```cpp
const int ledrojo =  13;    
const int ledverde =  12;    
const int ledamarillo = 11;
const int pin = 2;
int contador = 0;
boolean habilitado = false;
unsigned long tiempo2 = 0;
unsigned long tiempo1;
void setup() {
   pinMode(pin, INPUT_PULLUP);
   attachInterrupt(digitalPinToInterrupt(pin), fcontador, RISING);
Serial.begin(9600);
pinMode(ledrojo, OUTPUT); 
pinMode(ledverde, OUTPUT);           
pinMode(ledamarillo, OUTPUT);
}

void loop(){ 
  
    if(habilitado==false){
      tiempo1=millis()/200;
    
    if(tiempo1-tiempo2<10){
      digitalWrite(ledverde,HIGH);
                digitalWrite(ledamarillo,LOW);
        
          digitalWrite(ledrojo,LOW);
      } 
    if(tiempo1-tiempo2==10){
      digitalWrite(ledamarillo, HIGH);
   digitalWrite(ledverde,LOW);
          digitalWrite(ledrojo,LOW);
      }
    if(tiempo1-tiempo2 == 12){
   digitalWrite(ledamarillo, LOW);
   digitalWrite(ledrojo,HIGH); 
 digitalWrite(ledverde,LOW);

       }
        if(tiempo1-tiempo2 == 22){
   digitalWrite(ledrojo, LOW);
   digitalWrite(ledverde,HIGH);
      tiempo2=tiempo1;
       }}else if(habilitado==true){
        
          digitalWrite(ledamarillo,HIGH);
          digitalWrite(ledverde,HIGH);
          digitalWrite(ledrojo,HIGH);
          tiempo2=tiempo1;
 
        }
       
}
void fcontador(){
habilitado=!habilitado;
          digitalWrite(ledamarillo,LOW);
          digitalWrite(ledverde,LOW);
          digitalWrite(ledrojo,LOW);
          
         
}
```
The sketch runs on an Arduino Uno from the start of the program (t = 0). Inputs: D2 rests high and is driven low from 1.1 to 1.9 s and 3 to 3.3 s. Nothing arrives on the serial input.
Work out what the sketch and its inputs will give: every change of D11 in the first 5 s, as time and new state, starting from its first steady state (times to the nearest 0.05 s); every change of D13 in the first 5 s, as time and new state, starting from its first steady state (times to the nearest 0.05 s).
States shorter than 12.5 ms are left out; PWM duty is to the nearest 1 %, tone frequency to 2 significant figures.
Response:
0 s low; 1.9 s high; 3.3 s low; 3.8 s high; 4.2 s low
0 s low; 1.9 s high; 3.3 s low; 4.2 s high
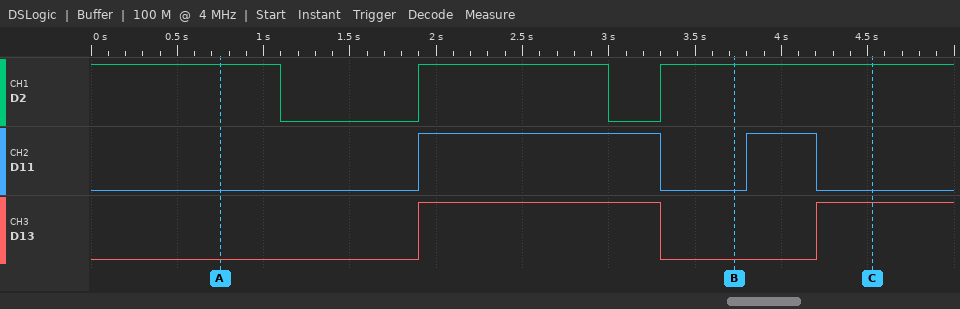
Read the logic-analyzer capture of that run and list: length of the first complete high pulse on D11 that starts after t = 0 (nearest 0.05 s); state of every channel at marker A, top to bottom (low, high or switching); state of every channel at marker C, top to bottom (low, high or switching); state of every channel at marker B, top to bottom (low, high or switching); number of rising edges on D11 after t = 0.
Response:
1.40 s
D2 high, D11 low, D13 low
D2 high, D11 low, D13 high
D2 high, D11 low, D13 low
2
